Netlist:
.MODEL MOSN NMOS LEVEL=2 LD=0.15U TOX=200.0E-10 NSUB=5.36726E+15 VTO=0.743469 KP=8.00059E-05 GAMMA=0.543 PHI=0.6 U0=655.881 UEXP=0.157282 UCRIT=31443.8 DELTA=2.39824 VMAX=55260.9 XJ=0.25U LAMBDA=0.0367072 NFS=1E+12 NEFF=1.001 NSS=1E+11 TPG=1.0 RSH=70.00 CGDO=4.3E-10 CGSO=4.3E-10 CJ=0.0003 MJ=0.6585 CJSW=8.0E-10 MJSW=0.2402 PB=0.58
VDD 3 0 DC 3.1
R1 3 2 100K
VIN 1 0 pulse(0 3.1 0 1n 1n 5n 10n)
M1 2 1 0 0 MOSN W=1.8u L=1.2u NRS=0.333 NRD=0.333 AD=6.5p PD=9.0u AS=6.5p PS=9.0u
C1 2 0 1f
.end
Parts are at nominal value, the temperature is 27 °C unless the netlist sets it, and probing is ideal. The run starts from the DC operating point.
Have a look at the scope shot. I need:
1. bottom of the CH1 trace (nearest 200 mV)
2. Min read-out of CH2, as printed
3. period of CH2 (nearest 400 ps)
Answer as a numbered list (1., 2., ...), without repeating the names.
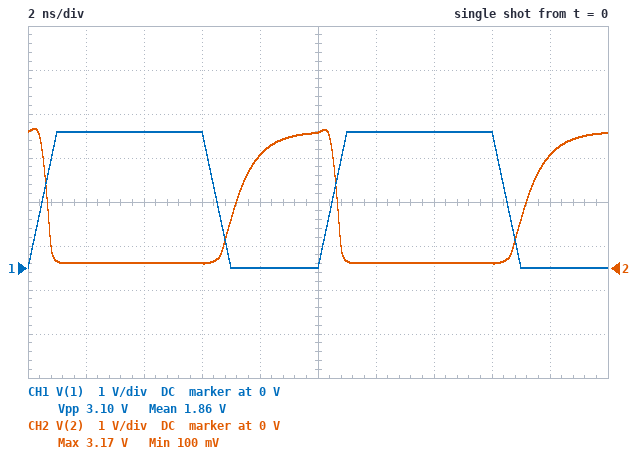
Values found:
1. 0 V
2. 100 mV
3. 10.0 ns
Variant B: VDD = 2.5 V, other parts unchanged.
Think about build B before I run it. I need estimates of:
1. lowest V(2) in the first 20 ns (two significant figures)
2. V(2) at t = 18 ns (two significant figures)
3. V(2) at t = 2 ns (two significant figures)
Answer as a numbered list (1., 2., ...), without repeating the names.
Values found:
1. 77 mV
2. 2.0 V
3. 95 mV
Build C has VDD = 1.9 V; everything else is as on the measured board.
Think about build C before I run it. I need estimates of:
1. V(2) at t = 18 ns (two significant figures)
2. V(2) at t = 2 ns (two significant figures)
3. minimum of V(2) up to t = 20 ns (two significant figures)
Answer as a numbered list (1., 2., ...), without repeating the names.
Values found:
1. 1.5 V
2. 72 mV
3. 53 mV
